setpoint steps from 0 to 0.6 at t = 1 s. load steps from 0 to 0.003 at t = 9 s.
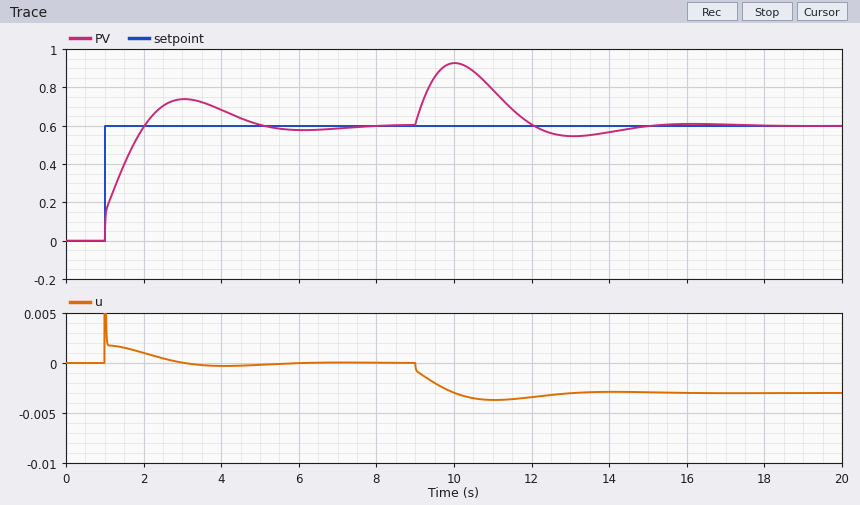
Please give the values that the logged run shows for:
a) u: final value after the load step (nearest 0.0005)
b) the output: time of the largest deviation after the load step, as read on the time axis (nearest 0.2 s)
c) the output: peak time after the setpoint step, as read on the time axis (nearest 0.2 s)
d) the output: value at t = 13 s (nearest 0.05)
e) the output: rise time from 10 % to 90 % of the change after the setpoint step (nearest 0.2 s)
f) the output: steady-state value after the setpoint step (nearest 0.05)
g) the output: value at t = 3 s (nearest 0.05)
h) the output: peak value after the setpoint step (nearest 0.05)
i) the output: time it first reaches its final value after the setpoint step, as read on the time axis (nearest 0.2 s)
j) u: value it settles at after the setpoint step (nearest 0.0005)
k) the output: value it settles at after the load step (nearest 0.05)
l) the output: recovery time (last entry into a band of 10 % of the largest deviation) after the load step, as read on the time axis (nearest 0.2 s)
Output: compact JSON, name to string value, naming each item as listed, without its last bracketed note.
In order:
{"u: final value after the load step": "-0.0030", "the output: time of the largest deviation after the load step, as read on the time axis": "10.0 s", "the output: peak time after the setpoint step, as read on the time axis": "3.0 s", "the output: value at t = 13 s": "0.55", "the output: rise time from 10 % to 90 % of the change after the setpoint step": "0.8 s", "the output: steady-state value after the setpoint step": "0.60", "the output: value at t = 3 s": "0.75", "the output: peak value after the setpoint step": "0.75", "the output: time it first reaches its final value after the setpoint step, as read on the time axis": "2.0 s", "u: value it settles at after the setpoint step": "0.0000", "the output: value it settles at after the load step": "0.60", "the output: recovery time (last entry into a band of 10 % of the largest deviation) after the load step, as read on the time axis": "14.0 s"}
